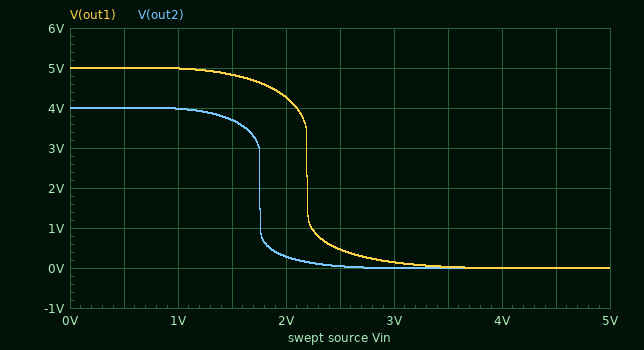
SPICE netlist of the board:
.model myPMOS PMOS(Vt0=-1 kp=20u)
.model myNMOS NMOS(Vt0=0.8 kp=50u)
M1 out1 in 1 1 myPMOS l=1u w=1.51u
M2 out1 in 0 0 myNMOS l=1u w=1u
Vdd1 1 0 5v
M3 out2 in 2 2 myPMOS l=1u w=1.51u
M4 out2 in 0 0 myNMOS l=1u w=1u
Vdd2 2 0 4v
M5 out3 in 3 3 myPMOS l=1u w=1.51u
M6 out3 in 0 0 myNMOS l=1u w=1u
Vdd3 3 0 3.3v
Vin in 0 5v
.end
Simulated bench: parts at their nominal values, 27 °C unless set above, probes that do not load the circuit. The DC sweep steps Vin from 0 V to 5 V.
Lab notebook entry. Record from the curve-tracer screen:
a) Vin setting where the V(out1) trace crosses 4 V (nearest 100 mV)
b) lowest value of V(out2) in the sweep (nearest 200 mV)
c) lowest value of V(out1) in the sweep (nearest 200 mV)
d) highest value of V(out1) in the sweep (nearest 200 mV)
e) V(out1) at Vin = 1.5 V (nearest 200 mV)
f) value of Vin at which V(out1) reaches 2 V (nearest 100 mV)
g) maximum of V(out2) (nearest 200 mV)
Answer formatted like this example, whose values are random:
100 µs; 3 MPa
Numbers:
2.1 V; 0 V; 0 V; 5.0 V; 4.8 V; 2.2 V; 4.0 V
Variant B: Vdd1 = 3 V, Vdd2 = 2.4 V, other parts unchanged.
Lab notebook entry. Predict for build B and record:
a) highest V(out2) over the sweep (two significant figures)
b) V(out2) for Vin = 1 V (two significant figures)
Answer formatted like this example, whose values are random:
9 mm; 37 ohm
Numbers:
2.4 V; 2.3 V
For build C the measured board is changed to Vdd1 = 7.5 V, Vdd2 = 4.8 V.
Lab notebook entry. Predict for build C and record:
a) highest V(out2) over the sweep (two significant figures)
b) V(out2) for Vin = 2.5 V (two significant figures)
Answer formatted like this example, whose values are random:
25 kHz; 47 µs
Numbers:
4.8 V; 330 mV
